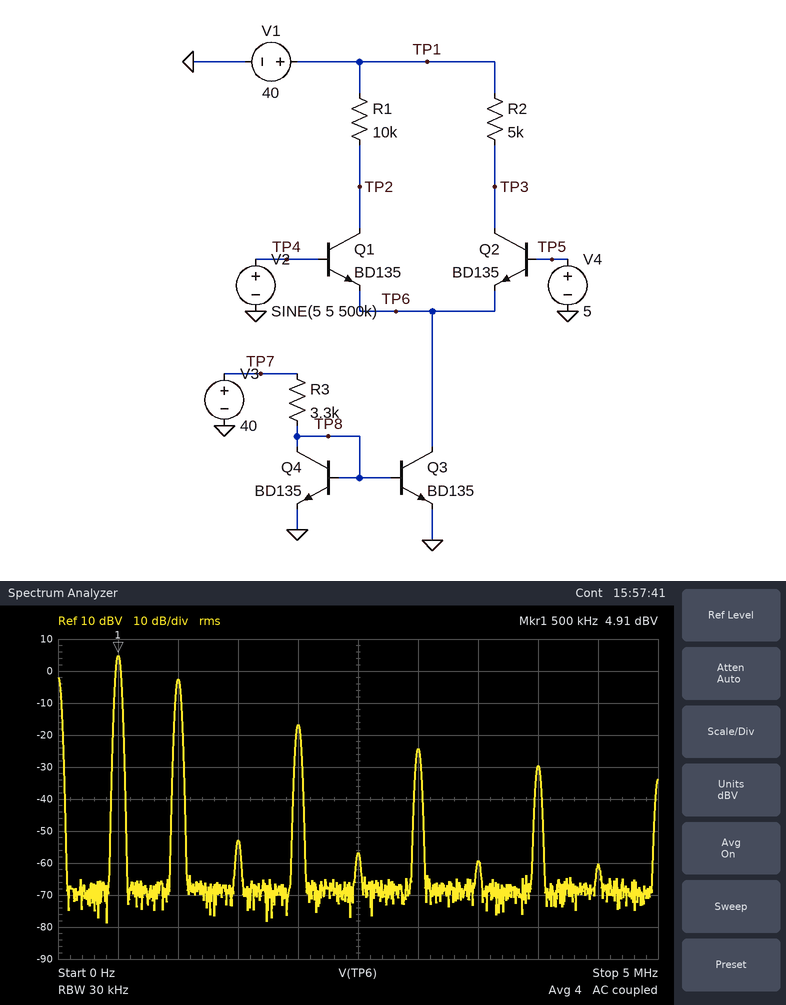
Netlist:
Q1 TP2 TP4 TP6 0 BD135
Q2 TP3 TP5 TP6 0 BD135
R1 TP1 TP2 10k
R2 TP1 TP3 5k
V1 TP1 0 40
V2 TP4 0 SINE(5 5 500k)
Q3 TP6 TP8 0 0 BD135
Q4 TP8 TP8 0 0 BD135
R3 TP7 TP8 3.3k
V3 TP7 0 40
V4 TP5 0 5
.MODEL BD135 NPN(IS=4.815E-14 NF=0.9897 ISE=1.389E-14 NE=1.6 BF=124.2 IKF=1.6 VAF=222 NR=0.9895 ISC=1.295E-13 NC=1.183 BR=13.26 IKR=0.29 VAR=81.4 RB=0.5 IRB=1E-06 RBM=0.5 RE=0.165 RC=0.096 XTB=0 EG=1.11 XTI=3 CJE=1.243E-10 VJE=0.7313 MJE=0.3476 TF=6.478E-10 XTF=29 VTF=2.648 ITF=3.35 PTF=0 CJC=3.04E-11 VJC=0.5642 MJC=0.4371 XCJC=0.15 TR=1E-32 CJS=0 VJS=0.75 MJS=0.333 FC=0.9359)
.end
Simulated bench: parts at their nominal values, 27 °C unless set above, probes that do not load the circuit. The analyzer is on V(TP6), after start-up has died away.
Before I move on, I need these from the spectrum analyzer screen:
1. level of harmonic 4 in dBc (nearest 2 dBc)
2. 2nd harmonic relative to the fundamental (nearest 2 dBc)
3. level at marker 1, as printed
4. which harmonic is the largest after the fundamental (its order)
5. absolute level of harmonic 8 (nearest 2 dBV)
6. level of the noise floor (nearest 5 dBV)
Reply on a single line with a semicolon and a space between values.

-22 dBc; -8 dBc; 4.91 dBV; 2; -30 dBV; -70 dBV
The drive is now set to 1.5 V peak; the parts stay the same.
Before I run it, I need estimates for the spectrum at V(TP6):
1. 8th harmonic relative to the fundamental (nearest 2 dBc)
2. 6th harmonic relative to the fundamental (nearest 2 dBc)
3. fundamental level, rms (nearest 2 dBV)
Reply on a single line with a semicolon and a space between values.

-36 dBc; -30 dBc; -6 dBV
